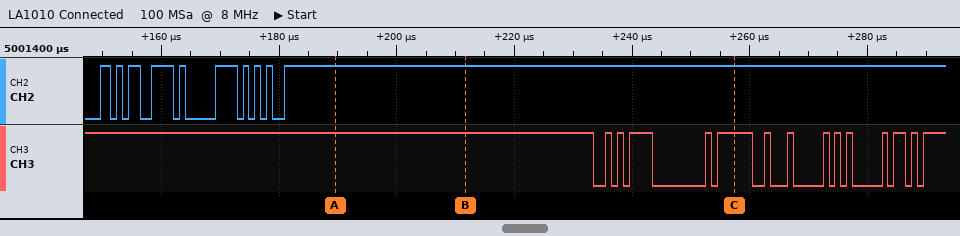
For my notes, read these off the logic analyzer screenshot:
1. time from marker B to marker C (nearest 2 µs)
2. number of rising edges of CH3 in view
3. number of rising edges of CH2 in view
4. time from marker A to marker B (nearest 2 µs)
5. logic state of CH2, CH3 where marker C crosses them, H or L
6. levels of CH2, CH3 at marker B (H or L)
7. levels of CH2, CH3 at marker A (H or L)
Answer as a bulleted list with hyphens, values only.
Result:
- 46 µs
- 14
- 10
- 22 µs
- CH2=H, CH3=H
- CH2=H, CH3=H
- CH2=H, CH3=H
